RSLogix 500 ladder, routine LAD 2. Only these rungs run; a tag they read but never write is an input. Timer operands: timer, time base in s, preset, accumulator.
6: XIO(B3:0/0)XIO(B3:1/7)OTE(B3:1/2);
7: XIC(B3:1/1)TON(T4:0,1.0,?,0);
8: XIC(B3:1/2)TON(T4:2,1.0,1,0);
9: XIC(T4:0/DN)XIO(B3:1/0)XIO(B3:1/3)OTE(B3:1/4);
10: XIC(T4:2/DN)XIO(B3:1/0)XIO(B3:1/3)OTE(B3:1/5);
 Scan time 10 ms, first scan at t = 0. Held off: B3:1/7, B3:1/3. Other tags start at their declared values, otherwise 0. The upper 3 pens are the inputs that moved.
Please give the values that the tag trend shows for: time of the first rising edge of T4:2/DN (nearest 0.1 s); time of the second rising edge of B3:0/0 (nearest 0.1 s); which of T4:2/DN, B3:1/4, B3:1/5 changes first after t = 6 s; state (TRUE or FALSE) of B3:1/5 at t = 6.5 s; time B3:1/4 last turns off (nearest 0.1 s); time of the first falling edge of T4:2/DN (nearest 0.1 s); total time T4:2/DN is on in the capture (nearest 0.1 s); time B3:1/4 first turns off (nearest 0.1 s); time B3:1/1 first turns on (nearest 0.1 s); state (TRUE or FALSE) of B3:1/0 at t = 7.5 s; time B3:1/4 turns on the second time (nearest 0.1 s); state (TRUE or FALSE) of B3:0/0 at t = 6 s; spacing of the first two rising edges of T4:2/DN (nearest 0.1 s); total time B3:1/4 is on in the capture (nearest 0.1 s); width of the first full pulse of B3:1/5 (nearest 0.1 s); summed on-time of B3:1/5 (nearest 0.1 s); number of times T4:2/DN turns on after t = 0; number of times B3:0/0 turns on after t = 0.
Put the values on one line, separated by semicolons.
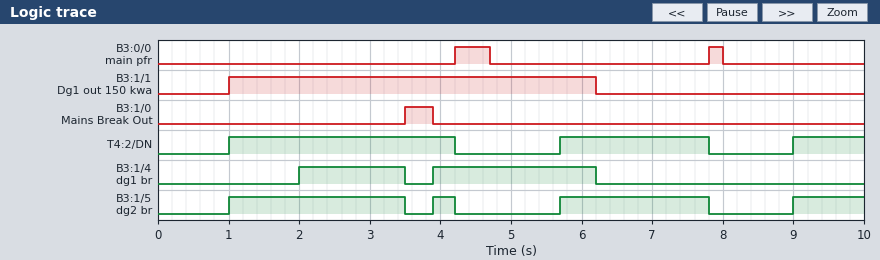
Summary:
1.0 s; 7.8 s; B3:1/4; TRUE; 6.2 s; 4.2 s; 6.3 s; 3.5 s; 1.0 s; FALSE; 3.9 s; FALSE; 4.7 s; 3.8 s; 2.5 s; 5.9 s; 3; 2
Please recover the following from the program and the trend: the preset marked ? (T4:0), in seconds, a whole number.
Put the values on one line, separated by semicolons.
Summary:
1 s
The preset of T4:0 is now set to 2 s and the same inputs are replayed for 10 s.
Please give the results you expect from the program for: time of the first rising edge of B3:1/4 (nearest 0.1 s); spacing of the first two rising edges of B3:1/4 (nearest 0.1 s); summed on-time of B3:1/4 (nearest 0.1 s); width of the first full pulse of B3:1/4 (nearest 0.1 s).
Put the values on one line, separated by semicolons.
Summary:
3.0 s; 0.9 s; 2.8 s; 0.5 s
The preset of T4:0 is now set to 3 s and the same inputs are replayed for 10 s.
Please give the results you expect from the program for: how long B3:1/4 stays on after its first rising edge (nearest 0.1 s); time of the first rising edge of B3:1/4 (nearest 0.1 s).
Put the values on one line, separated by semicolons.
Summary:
2.2 s; 4.0 s
